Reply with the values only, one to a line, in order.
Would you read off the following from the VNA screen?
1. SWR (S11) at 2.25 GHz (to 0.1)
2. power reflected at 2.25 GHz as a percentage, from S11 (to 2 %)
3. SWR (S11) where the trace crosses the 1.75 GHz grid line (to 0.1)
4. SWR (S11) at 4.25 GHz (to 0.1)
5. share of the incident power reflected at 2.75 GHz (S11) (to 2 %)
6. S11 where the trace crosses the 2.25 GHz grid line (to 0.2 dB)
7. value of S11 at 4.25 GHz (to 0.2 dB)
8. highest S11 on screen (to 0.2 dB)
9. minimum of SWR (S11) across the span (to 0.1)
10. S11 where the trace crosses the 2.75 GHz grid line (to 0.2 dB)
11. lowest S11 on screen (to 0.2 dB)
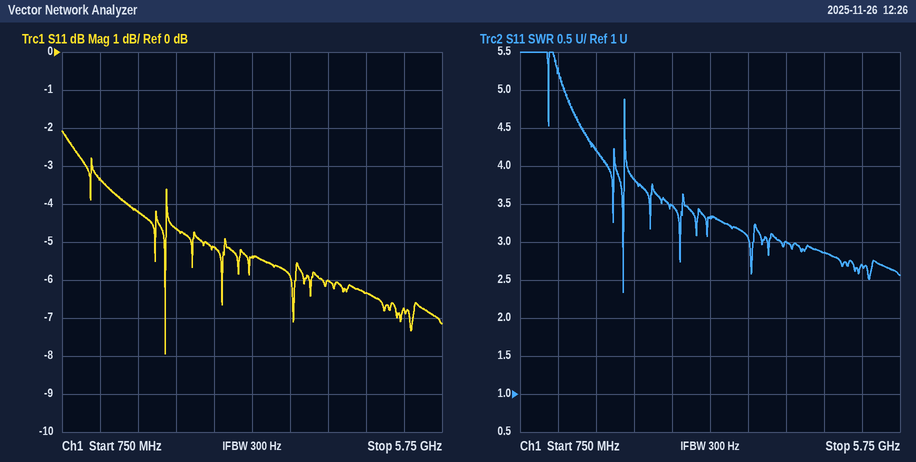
3.8
34 %
4.2
3.0
30 %
-4.6 dB
-6.0 dB
-2.0 dB
2.3
-5.2 dB
-8.0 dB
